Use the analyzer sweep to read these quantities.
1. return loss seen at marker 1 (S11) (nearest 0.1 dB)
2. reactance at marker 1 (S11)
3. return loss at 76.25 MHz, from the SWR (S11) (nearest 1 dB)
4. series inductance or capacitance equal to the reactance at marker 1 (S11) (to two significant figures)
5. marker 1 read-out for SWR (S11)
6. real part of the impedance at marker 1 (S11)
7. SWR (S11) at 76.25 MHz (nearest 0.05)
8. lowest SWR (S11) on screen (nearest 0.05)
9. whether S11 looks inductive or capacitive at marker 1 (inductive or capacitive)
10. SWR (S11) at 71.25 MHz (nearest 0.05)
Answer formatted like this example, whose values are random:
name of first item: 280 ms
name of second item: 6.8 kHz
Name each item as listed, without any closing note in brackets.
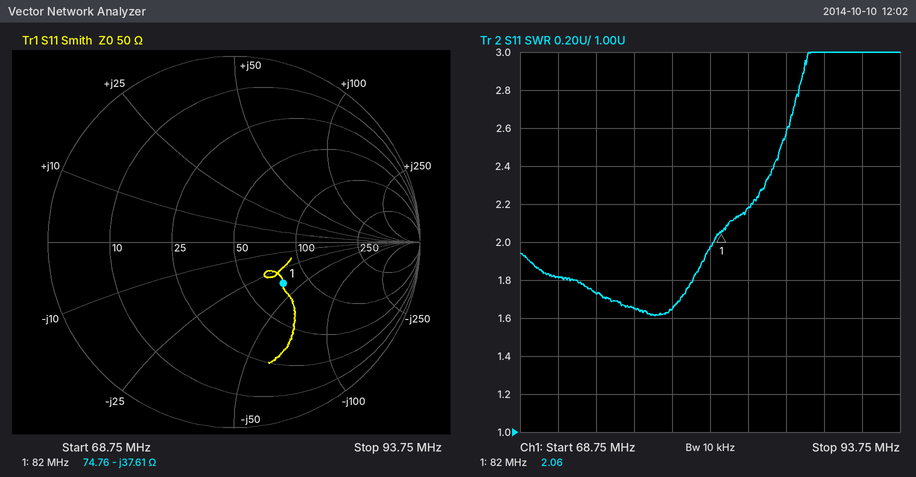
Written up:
return loss seen at marker 1 (S11): 9.2 dB
reactance at marker 1: -37.61 Ω
return loss at 76.25 MHz, from the SWR (S11): 12 dB
series inductance or capacitance equal to the reactance at marker 1 (S11): 52 pF
marker 1 read-out for SWR: 2.06
real part of the impedance at marker 1: 74.76 Ω
SWR (S11) at 76.25 MHz: 1.65
lowest SWR (S11) on screen: 1.60
whether S11 looks inductive or capacitive at marker 1: capacitive
SWR (S11) at 71.25 MHz: 1.80
